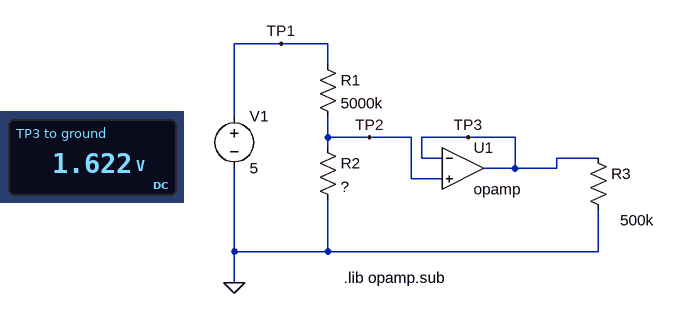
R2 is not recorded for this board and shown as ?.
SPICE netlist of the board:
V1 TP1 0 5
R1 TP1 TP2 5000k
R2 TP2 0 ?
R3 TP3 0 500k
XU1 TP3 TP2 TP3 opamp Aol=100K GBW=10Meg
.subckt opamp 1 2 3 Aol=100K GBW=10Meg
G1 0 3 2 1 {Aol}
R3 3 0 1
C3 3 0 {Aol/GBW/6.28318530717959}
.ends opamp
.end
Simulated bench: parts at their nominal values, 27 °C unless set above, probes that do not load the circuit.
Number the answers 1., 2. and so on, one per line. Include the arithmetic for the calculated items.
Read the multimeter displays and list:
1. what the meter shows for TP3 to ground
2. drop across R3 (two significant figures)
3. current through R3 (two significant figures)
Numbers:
1. 1.622 V
2. 1.622 V = 1.6 V
3. (1.622 V) / 500 kΩ = 3.2 µA
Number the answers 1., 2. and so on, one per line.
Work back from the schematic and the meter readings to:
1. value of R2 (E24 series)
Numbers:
1. 2.4 MΩ
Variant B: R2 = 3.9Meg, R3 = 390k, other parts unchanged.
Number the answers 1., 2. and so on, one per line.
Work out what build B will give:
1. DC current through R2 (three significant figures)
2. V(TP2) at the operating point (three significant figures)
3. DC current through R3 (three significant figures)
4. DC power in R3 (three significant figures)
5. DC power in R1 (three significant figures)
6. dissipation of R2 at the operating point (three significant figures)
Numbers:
1. 562 nA
2. 2.19 V
3. 5.62 µA
4. 12.3 µW
5. 1.58 µW
6. 1.23 µW
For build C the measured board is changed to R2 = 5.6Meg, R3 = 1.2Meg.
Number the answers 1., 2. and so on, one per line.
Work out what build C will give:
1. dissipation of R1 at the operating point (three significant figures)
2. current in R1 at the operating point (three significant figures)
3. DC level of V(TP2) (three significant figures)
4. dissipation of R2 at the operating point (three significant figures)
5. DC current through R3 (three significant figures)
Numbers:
1. 1.11 µW
2. 472 nA
3. 2.64 V
4. 1.25 µW
5. 2.20 µA
